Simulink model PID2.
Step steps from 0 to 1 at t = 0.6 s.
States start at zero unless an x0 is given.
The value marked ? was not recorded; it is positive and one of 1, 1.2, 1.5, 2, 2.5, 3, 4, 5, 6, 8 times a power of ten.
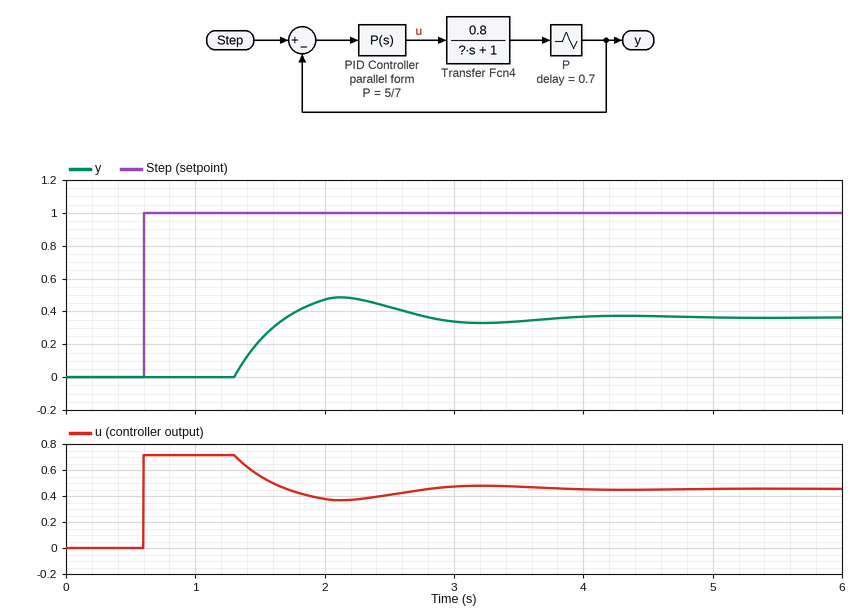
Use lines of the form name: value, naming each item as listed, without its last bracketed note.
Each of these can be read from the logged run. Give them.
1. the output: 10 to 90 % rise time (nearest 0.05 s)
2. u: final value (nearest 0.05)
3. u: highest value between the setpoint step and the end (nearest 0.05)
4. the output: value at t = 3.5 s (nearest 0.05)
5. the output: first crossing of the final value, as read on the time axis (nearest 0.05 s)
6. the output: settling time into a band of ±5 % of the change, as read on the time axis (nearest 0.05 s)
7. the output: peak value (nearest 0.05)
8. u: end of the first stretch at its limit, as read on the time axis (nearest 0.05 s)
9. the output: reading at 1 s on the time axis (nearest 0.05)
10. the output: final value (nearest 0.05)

the output: 10 to 90 % rise time: 0.30 s
u: final value: 0.45
u: highest value between the setpoint step and the end: 0.70
the output: value at t = 3.5 s: 0.35
the output: first crossing of the final value, as read on the time axis: 1.70 s
the output: settling time into a band of ±5 % of the change, as read on the time axis: 3.60 s
the output: peak value: 0.50
u: end of the first stretch at its limit, as read on the time axis: 1.30 s
the output: reading at 1 s on the time axis: 0.00
the output: final value: 0.35
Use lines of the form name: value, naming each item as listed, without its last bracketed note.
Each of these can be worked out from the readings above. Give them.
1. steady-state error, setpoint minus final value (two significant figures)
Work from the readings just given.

steady-state error, setpoint minus final value: 0.65
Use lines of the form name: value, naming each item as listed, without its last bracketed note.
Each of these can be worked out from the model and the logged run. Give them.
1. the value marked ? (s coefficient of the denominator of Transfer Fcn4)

the value marked ?: 0.4
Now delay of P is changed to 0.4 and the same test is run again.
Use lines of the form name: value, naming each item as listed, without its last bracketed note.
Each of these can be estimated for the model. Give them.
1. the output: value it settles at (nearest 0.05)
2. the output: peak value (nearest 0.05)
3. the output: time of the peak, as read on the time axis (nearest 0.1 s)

the output: value it settles at: 0.35
the output: peak value: 0.40
the output: time of the peak, as read on the time axis: 1.7 s
